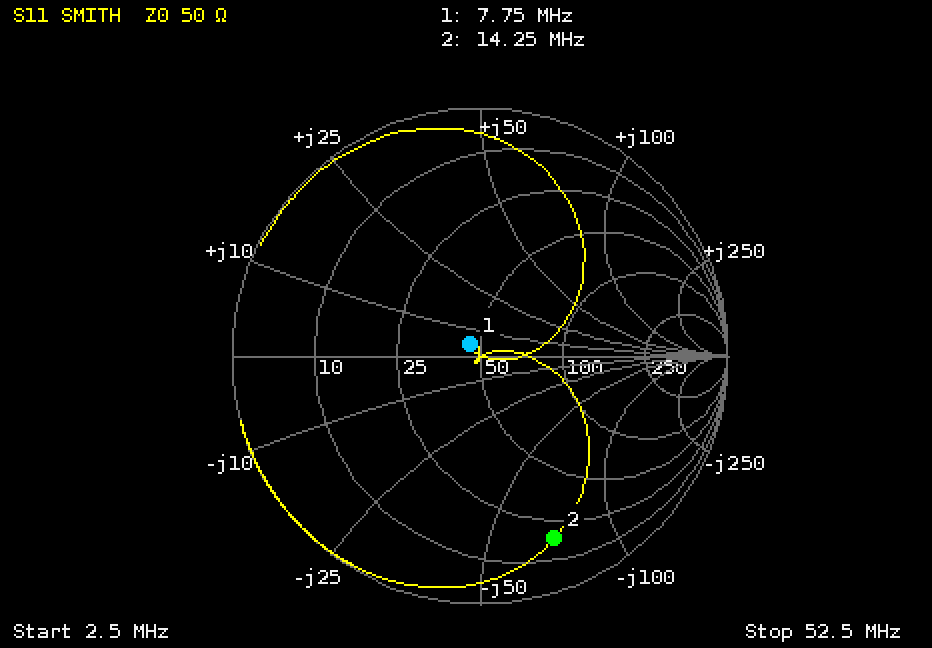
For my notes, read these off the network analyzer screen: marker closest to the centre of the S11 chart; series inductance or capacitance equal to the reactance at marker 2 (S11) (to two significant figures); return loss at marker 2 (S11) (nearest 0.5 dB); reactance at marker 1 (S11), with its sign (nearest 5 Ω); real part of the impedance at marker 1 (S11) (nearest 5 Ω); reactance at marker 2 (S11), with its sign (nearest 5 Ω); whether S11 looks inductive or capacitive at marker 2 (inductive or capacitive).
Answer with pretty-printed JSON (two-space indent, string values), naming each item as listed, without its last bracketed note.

{
  "marker closest to the centre of the S11 chart": "marker 1",
  "series inductance or capacitance equal to the reactance at marker 2 (S11)": "160 pF",
  "return loss at marker 2 (S11)": "2.0 dB",
  "reactance at marker 1 (S11), with its sign": "+5 Ω",
  "real part of the impedance at marker 1 (S11)": "45 Ω",
  "reactance at marker 2 (S11), with its sign": "-70 Ω",
  "whether S11 looks inductive or capacitive at marker 2": "capacitive"
}
